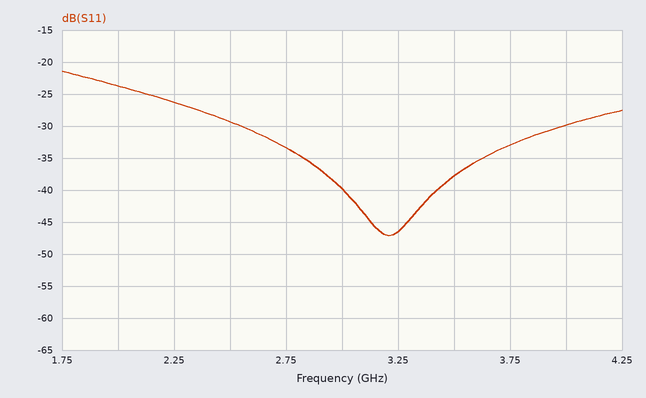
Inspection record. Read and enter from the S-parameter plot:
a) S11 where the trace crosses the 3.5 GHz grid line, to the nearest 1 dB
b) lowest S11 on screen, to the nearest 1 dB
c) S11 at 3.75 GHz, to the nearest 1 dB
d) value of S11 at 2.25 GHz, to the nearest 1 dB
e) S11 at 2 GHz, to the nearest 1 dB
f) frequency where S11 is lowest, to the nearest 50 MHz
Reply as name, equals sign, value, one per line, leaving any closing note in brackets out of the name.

S11 where the trace crosses the 3.5 GHz grid line, to the nearest 1 dB = -38 dB
lowest S11 on screen, to the nearest 1 dB = -47 dB
S11 at 3.75 GHz, to the nearest 1 dB = -33 dB
value of S11 at 2.25 GHz, to the nearest 1 dB = -26 dB
S11 at 2 GHz, to the nearest 1 dB = -24 dB
frequency where S11 is lowest, to the nearest 50 MHz = 3.20 GHz
